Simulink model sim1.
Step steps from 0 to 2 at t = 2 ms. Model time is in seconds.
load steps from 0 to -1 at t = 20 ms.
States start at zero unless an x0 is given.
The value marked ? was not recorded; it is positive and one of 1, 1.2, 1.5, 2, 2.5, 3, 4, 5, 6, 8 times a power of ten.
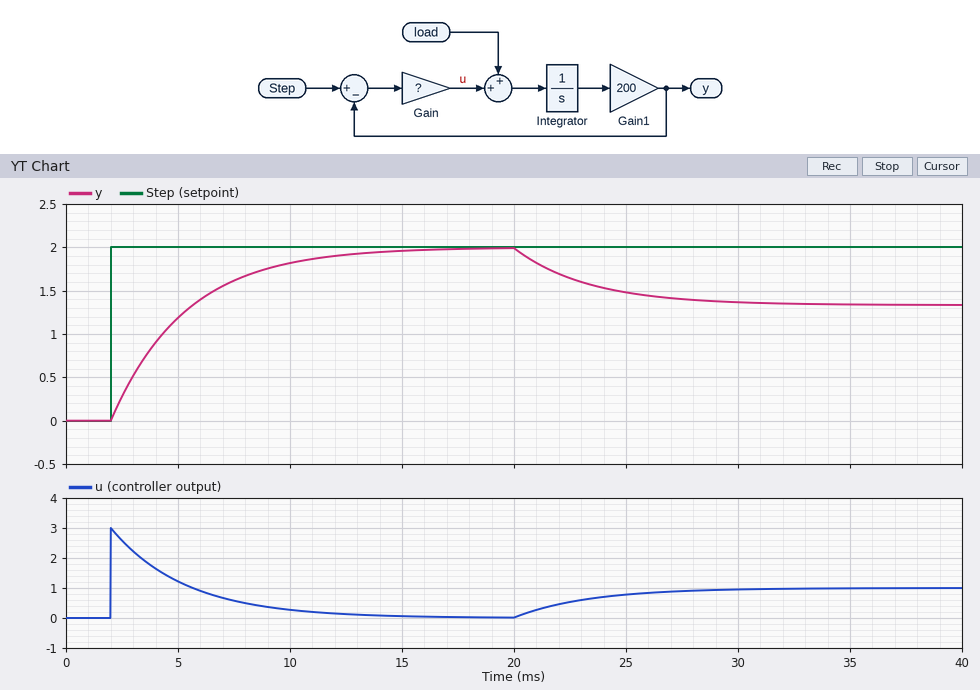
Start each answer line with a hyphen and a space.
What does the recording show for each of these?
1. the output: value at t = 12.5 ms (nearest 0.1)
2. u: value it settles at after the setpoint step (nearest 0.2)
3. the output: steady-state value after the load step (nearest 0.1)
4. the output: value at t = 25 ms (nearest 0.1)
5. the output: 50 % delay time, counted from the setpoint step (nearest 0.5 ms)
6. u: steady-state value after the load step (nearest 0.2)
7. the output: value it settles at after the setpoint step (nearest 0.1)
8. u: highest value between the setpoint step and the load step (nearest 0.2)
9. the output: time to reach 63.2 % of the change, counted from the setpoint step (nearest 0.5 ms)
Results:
- 1.9
- 0.0
- 1.3
- 1.5
- 2.5 ms
- 1.0
- 2.0
- 3.0
- 3.5 ms
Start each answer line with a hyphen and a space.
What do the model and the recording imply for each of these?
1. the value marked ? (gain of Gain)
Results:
- 1.5
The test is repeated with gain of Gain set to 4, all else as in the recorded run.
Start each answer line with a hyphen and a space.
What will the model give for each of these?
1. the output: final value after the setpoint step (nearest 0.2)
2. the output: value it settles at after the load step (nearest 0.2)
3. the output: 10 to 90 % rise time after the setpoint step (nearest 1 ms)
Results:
- 2.0
- 1.8
- 3 ms
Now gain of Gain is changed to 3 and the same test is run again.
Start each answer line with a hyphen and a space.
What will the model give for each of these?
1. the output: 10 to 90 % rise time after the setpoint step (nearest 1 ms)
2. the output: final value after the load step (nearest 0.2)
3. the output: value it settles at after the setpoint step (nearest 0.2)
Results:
- 4 ms
- 1.6
- 2.0
